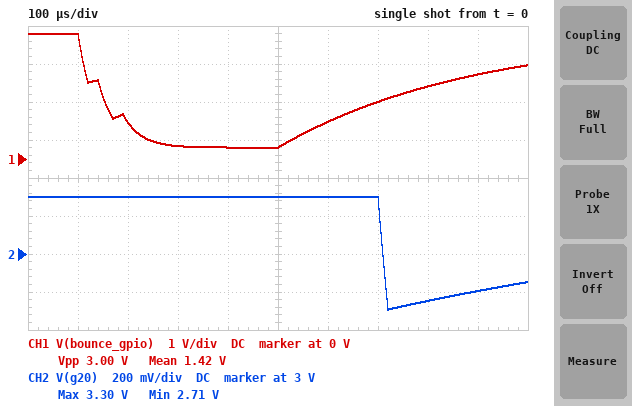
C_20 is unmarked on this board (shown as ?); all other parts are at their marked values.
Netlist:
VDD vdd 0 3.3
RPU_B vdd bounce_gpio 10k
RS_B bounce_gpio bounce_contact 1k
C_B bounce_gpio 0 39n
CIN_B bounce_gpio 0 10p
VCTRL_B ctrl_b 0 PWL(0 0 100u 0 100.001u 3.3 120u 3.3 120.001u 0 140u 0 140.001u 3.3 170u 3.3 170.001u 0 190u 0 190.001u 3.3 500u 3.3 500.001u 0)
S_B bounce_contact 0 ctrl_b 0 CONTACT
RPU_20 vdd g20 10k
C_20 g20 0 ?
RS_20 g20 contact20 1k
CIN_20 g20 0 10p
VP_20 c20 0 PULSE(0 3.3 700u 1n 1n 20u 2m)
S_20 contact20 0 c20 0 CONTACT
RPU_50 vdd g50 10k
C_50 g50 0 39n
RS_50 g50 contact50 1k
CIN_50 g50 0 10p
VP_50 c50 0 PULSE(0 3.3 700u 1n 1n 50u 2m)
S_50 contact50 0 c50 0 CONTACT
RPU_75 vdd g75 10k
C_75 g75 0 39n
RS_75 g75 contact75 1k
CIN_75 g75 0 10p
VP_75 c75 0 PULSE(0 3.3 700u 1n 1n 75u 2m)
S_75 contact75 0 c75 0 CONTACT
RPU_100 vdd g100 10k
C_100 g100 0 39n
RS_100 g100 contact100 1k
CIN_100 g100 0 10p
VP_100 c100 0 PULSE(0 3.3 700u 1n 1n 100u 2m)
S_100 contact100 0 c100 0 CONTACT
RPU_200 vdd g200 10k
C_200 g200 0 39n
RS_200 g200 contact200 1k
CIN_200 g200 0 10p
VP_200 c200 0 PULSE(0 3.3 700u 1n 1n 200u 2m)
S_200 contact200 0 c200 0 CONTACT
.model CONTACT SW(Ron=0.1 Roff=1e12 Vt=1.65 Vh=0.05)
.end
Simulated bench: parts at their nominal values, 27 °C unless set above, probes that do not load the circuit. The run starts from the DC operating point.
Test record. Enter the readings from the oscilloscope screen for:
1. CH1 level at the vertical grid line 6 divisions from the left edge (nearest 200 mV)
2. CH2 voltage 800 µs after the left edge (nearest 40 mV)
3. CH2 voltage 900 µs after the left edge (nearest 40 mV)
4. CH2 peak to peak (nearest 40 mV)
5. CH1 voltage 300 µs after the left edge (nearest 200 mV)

1.0 V
2.76 V
2.80 V
600 mV
400 mV
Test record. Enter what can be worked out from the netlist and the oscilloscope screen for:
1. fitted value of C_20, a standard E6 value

100 nF
